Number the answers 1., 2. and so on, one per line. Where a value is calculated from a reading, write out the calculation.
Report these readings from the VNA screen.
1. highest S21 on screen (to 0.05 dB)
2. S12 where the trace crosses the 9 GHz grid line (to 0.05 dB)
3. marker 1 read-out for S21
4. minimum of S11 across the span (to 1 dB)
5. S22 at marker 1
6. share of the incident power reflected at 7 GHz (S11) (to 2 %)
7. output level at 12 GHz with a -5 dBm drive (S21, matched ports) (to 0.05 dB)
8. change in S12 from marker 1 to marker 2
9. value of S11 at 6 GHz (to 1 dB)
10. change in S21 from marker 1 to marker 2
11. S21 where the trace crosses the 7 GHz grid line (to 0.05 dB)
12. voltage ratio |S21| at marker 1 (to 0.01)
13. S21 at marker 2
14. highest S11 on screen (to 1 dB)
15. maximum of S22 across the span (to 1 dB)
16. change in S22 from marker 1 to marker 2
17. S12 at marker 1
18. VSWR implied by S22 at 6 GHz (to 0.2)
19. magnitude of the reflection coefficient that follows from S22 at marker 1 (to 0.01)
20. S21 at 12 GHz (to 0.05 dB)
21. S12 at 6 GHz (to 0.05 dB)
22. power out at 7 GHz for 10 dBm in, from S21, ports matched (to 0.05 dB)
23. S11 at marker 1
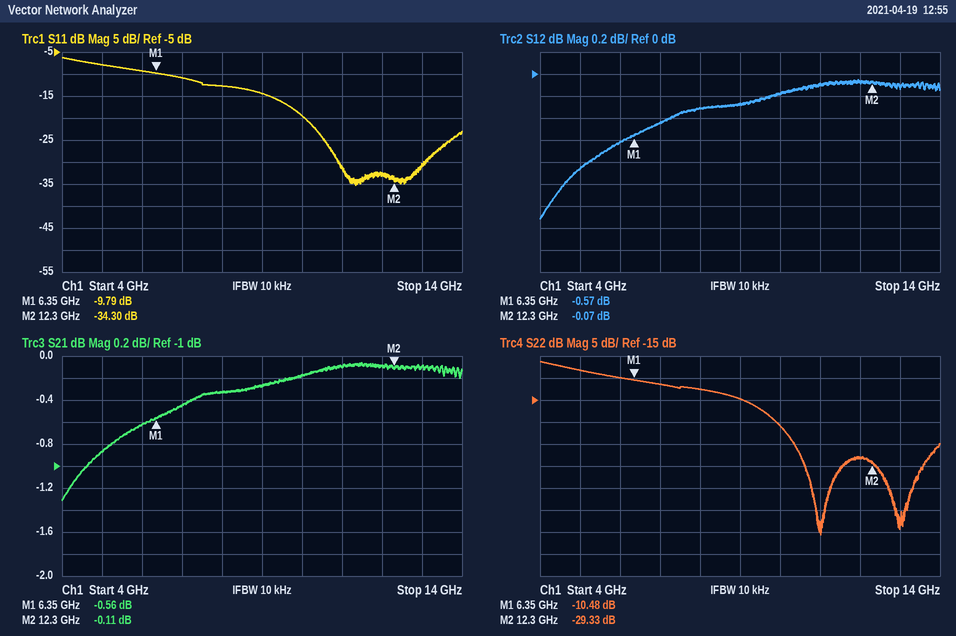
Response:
1. -0.05 dB
2. -0.25 dB
3. -0.56 dB
4. -35 dB
5. -10.48 dB
6. 10^(-11/10) ≈ 8 %
7. -5 dBm + (-0.10 dB) = -5.10 dBm
8. -0.07 − (-0.57) = 0.50 dB
9. -9 dB
10. -0.11 − (-0.56) = 0.45 dB
11. -0.45 dB
12. 10^(-0.56/20) ≈ 0.94
13. -0.11 dB
14. -6 dB
15. -6 dB
16. -29.33 − (-10.48) = -18.85 dB
17. -0.57 dB
18. |Γ| = 10^(-10/20) = 0.3162; VSWR = (1 + 0.3162)/(1 − 0.3162) ≈ 1.92, so 2.0 to the nearest 0.2
19. 10^(-10.48/20) ≈ 0.30
20. -0.10 dB
21. -0.60 dB
22. 10 dBm + (-0.45 dB) = 9.55 dBm
23. -9.79 dB
